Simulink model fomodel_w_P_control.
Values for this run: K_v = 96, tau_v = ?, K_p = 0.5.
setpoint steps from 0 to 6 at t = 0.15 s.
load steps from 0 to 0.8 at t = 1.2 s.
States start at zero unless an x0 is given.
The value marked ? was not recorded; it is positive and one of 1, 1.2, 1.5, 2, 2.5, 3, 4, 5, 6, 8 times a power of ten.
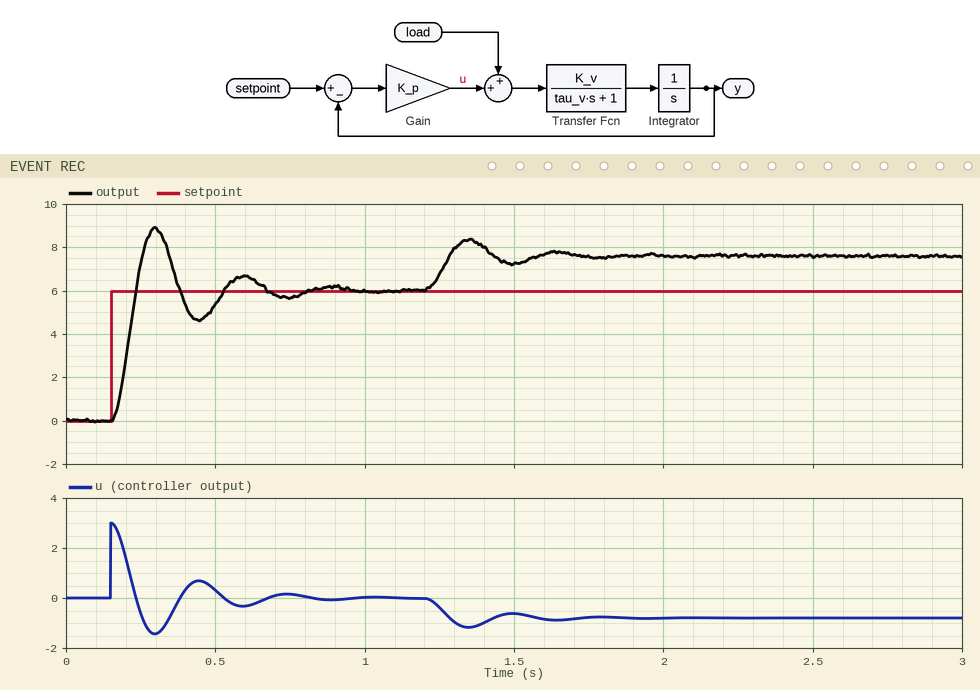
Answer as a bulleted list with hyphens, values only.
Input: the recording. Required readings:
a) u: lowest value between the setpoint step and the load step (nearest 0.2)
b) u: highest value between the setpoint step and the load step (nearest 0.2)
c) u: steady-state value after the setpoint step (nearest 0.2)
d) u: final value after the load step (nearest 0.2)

- -1.4
- 3.0
- 0.0
- -0.8
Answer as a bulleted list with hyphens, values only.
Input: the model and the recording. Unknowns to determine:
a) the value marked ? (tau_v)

- 0.1
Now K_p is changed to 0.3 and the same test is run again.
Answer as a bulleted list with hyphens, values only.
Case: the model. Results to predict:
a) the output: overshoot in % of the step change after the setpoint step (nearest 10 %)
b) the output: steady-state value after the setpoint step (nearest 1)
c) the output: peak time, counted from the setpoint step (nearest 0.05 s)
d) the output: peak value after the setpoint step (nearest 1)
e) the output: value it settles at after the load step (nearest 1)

- 40 %
- 6
- 0.20 s
- 8
- 9
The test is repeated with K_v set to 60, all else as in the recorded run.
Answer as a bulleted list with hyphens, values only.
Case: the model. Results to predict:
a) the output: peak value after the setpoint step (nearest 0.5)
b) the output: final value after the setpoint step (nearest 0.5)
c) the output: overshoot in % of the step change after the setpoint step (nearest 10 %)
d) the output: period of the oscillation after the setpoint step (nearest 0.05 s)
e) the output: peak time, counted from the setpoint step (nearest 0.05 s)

- 8.5
- 6.0
- 40 %
- 0.40 s
- 0.20 s
